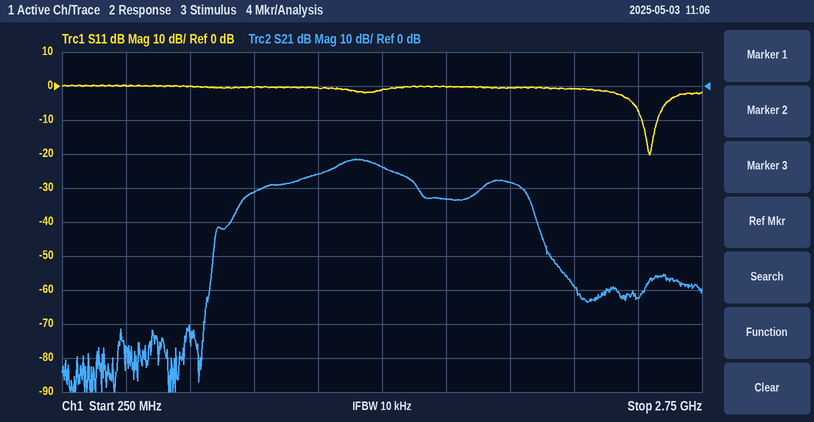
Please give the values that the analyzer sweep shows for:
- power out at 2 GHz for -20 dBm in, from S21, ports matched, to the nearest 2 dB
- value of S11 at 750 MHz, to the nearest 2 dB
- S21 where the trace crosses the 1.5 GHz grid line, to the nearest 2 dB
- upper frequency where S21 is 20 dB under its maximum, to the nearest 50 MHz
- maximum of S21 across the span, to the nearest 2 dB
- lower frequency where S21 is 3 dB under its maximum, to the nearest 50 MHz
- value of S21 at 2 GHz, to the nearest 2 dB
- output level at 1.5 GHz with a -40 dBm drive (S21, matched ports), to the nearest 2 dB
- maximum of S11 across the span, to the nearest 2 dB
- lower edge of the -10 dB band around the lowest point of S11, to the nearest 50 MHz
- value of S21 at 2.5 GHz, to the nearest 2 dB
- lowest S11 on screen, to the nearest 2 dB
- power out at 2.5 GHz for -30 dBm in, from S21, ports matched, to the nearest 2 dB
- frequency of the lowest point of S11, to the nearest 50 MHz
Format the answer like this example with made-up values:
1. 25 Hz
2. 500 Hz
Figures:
1. -48 dBm
2. 0 dB
3. -24 dB
4. 2.10 GHz
5. -22 dB
6. 1.30 GHz
7. -28 dB
8. -64 dBm
9. 0 dB
10. 2.50 GHz
11. -62 dB
12. -20 dB
13. -92 dBm
14. 2.55 GHz
